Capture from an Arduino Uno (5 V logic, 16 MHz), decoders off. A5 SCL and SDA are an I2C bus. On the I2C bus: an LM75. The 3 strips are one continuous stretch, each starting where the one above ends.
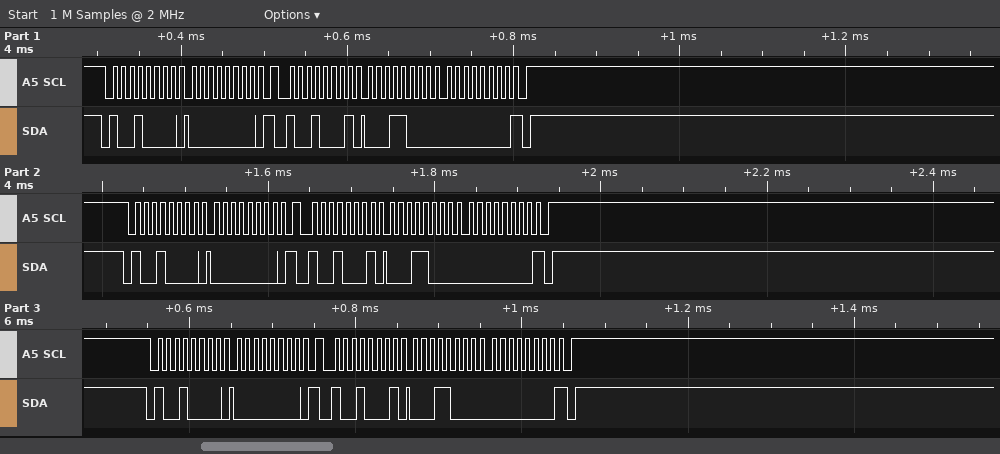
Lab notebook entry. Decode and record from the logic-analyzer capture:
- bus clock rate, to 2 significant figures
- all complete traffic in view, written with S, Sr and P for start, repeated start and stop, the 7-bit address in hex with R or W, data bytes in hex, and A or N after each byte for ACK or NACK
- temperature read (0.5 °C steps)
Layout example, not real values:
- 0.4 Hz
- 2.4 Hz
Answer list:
- 100 kHz
- S 48W A 00 A Sr 48R A 18 A 00 N P S 48W A 00 A Sr 48R A 18 A 00 N P S 48W A 00 A Sr 48R A 18 A 00 N P
- 24.0 °C
